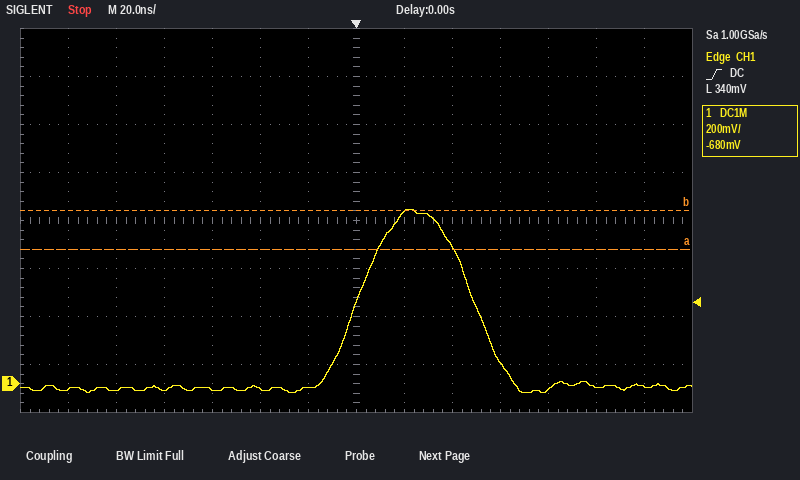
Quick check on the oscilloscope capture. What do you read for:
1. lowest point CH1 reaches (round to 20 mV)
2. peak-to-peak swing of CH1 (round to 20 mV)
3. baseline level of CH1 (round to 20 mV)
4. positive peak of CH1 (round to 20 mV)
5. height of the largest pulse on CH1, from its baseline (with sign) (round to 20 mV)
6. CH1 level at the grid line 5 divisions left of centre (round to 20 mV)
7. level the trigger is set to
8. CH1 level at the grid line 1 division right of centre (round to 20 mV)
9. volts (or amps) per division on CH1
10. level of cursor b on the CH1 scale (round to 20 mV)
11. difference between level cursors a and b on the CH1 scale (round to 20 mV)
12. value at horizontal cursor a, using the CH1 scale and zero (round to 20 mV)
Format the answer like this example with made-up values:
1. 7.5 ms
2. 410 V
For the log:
1. -40 mV
2. 760 mV
3. -20 mV
4. 720 mV
5. +740 mV
6. -20 mV
7. 340 mV
8. 720 mV
9. 200 mV
10. 720 mV
11. 160 mV
12. 560 mV
